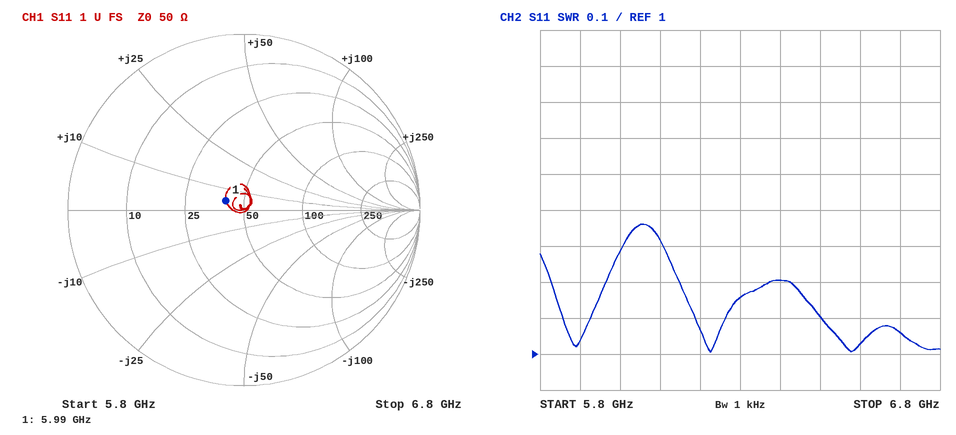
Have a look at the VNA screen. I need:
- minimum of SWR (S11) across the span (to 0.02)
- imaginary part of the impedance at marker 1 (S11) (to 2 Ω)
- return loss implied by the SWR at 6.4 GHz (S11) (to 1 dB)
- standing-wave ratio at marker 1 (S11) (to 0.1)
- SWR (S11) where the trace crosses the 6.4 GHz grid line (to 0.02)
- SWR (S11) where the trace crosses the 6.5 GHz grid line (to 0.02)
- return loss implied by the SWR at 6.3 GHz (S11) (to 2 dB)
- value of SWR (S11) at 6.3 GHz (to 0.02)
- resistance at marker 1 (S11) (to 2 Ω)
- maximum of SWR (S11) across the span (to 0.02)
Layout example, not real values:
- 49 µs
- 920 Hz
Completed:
- 1.00
- +4 Ω
- 21 dB
- 1.3
- 1.20
- 1.10
- 22 dB
- 1.16
- 40 Ω
- 1.36
